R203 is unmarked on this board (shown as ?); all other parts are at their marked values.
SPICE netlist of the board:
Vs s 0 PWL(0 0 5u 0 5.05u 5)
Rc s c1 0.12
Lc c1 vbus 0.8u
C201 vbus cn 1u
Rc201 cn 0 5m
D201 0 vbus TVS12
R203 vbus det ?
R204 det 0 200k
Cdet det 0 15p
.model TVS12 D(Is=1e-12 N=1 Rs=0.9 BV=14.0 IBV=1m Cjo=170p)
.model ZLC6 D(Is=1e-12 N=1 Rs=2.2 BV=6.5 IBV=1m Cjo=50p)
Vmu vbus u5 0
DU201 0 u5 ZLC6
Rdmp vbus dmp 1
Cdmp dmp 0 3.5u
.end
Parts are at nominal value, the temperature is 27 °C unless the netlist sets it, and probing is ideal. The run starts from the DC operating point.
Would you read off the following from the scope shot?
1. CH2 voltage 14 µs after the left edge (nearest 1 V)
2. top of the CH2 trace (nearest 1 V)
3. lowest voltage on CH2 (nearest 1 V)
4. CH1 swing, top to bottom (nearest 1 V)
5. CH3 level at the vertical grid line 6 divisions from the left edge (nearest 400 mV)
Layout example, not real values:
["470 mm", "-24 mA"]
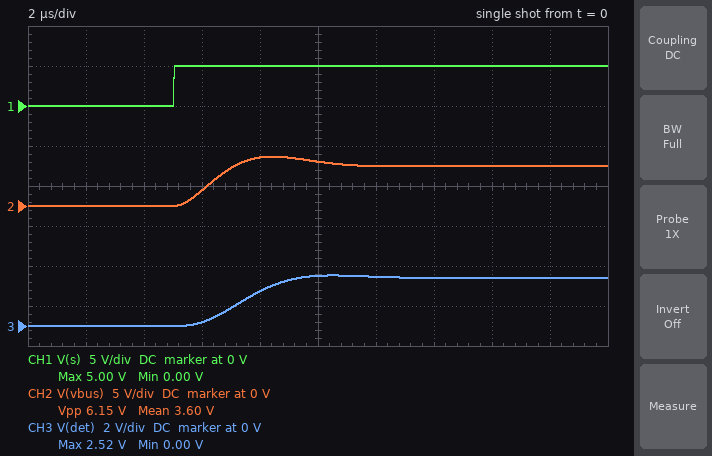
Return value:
["5 V", "6 V", "0 V", "5 V", "2.4 V"]
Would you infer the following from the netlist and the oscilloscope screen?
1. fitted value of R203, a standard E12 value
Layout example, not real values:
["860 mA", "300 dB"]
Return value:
["220 kΩ"]
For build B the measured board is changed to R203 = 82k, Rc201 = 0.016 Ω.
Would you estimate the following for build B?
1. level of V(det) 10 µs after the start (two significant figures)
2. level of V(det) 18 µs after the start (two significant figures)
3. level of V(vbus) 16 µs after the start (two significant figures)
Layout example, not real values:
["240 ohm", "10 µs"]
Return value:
["4.1 V", "3.6 V", "5.0 V"]
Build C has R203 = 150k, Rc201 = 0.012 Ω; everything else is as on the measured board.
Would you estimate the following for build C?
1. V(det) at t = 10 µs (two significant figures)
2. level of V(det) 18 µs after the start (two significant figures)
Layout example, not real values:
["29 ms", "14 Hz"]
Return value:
["3.1 V", "2.9 V"]
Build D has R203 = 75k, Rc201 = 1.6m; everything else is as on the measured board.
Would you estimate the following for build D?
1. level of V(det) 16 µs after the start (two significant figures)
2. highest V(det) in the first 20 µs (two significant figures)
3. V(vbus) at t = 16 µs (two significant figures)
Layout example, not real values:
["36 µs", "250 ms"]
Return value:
["3.7 V", "4.2 V", "5.0 V"]
